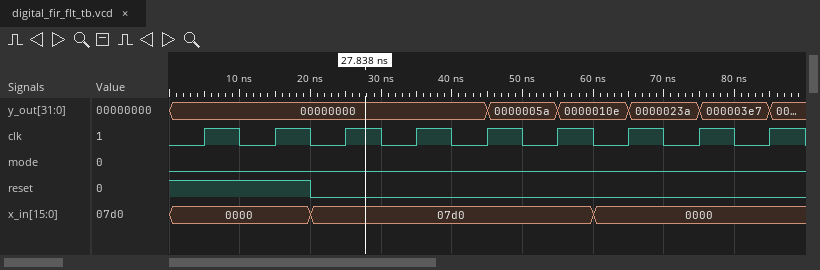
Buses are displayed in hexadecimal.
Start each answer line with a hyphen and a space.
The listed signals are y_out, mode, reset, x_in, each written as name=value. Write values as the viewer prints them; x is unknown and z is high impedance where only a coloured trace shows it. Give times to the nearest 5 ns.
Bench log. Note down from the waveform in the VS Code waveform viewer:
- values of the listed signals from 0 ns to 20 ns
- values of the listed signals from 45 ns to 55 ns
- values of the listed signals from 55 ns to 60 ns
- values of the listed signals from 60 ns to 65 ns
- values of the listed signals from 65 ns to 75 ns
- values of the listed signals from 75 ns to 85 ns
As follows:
- y_out=00000000, mode=0, reset=1, x_in=0000
- y_out=0000005a, mode=0, reset=0, x_in=07d0
- y_out=0000010e, mode=0, reset=0, x_in=07d0
- y_out=0000010e, mode=0, reset=0, x_in=0000
- y_out=0000023a, mode=0, reset=0, x_in=0000
- y_out=000003e7, mode=0, reset=0, x_in=0000
